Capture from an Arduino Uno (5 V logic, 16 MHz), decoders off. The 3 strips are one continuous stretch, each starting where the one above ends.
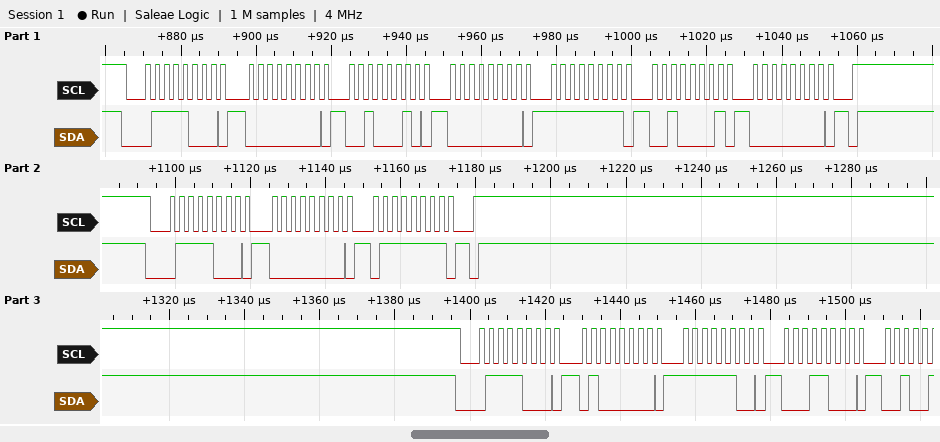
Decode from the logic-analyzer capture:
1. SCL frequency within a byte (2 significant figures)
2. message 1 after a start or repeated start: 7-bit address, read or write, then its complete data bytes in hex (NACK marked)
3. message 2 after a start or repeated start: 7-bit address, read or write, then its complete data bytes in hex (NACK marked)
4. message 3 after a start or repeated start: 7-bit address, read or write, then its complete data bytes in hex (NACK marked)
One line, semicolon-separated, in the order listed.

400 kHz; 0x3C write: 00 22 00 FF 21 00; 0x3C write: 00 7F; 0x3C write: 40 FC 18
